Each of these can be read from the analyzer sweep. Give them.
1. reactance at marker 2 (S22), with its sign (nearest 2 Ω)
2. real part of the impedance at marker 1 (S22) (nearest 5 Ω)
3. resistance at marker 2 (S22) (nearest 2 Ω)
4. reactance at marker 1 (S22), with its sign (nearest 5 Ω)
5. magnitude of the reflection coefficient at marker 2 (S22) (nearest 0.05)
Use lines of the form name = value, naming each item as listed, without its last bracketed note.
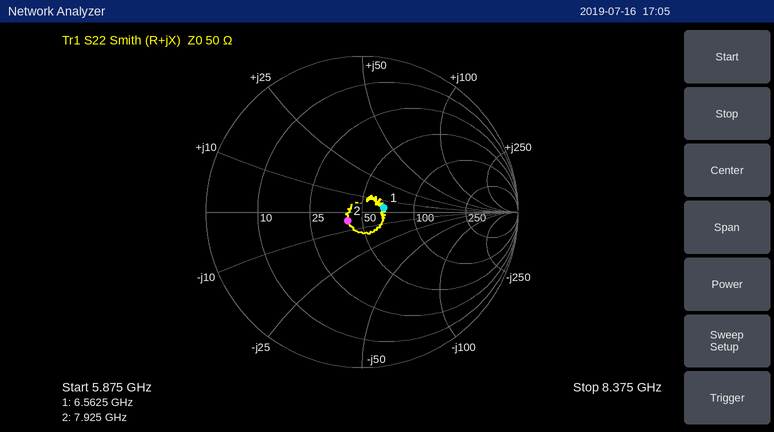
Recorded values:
reactance at marker 2 (S22), with its sign = -4 Ω
real part of the impedance at marker 1 (S22) = 65 Ω
resistance at marker 2 (S22) = 42 Ω
reactance at marker 1 (S22), with its sign = +5 Ω
magnitude of the reflection coefficient at marker 2 (S22) = 0.10
